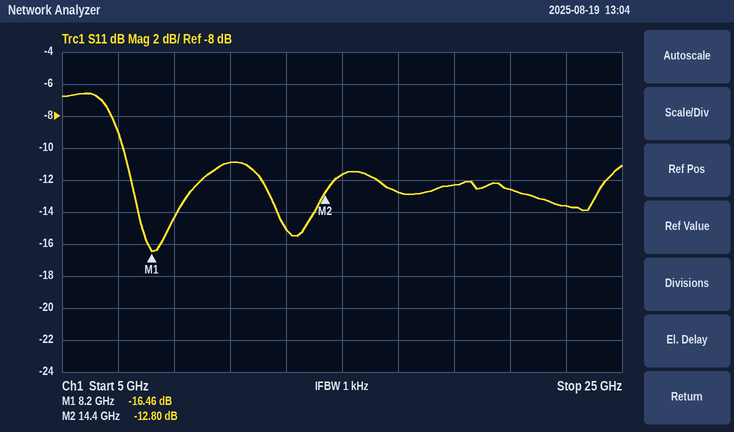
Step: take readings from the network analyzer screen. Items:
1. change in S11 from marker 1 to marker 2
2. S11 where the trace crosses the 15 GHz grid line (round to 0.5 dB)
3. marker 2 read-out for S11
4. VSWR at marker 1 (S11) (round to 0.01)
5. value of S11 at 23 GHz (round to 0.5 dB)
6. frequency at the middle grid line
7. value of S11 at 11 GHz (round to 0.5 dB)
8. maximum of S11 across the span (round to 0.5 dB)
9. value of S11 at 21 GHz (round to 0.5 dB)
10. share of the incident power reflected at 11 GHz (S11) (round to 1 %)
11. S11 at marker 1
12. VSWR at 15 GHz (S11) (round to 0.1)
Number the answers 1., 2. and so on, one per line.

1. 3.66 dB
2. -11.5 dB
3. -12.80 dB
4. 1.35
5. -13.5 dB
6. 15 GHz
7. -11.0 dB
8. -6.5 dB
9. -12.5 dB
10. 8 %
11. -16.46 dB
12. 1.7
